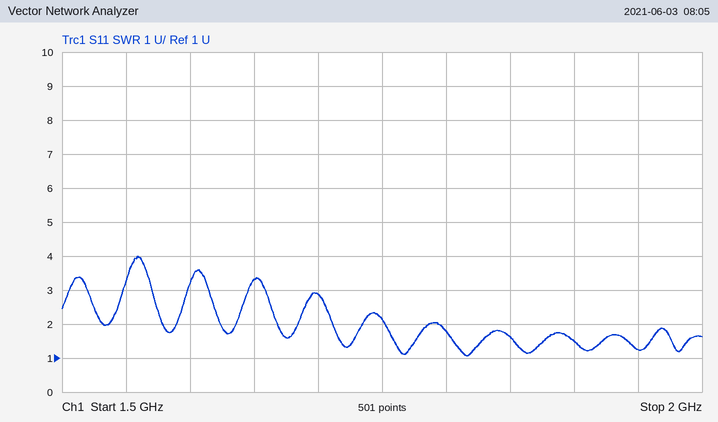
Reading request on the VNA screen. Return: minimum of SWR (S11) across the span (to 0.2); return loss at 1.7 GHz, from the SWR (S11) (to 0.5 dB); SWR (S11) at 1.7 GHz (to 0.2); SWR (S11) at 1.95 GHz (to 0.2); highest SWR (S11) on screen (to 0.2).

1.0
6.5 dB
2.8
1.2
4.0
